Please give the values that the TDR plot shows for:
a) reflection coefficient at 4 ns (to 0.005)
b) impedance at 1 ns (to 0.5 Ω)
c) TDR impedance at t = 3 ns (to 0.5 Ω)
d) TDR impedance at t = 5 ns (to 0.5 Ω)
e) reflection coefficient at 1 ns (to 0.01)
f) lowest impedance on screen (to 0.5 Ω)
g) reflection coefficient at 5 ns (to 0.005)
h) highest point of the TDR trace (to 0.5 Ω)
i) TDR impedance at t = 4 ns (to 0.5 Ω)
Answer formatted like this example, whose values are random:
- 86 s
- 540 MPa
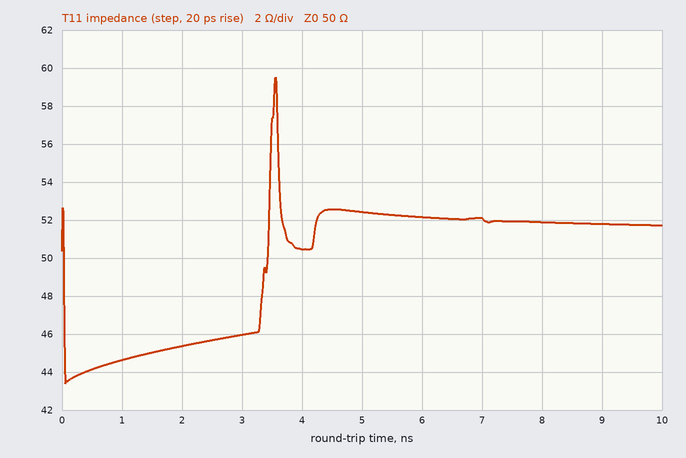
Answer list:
- +0.005
- 44.5 Ω
- 46.0 Ω
- 52.5 Ω
- -0.06
- 43.5 Ω
- +0.025
- 59.5 Ω
- 50.5 Ω
